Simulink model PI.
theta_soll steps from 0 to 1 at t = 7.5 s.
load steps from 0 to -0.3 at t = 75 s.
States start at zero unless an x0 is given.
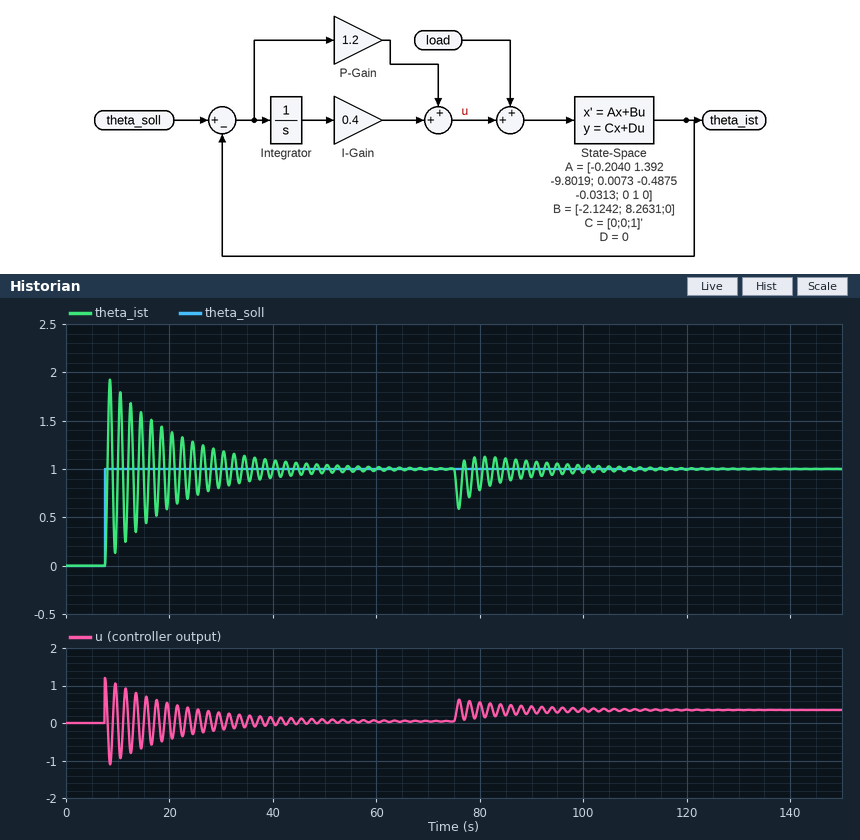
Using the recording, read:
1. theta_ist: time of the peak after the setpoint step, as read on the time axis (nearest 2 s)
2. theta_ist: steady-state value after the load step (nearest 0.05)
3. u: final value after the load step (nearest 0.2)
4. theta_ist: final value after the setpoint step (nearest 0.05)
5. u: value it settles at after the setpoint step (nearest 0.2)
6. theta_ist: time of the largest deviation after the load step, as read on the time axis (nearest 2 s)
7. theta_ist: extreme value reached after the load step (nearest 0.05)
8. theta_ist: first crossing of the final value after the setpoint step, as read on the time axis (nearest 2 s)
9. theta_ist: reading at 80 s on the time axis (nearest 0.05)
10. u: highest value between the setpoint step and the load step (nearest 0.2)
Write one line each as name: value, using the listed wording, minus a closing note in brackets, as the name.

theta_ist: time of the peak after the setpoint step, as read on the time axis: 8 s
theta_ist: steady-state value after the load step: 1.00
u: final value after the load step: 0.4
theta_ist: final value after the setpoint step: 1.00
u: value it settles at after the setpoint step: 0.0
theta_ist: time of the largest deviation after the load step, as read on the time axis: 76 s
theta_ist: extreme value reached after the load step: 0.60
theta_ist: first crossing of the final value after the setpoint step, as read on the time axis: 8 s
theta_ist: reading at 80 s on the time axis: 0.80
u: highest value between the setpoint step and the load step: 1.2
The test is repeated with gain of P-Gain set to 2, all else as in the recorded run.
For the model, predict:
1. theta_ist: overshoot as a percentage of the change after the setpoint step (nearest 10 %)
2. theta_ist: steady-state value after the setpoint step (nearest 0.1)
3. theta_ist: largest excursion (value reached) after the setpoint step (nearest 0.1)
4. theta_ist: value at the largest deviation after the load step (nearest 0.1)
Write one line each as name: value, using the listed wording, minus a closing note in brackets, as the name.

theta_ist: overshoot as a percentage of the change after the setpoint step: 90 %
theta_ist: steady-state value after the setpoint step: 1.0
theta_ist: largest excursion (value reached) after the setpoint step: 1.9
theta_ist: value at the largest deviation after the load step: 0.7
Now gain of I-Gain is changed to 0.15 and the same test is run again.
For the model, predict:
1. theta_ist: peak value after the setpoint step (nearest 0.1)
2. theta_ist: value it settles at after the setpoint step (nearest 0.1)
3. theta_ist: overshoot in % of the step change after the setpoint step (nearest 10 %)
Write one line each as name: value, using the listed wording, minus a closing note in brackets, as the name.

theta_ist: peak value after the setpoint step: 1.8
theta_ist: value it settles at after the setpoint step: 1.0
theta_ist: overshoot in % of the step change after the setpoint step: 80 %
